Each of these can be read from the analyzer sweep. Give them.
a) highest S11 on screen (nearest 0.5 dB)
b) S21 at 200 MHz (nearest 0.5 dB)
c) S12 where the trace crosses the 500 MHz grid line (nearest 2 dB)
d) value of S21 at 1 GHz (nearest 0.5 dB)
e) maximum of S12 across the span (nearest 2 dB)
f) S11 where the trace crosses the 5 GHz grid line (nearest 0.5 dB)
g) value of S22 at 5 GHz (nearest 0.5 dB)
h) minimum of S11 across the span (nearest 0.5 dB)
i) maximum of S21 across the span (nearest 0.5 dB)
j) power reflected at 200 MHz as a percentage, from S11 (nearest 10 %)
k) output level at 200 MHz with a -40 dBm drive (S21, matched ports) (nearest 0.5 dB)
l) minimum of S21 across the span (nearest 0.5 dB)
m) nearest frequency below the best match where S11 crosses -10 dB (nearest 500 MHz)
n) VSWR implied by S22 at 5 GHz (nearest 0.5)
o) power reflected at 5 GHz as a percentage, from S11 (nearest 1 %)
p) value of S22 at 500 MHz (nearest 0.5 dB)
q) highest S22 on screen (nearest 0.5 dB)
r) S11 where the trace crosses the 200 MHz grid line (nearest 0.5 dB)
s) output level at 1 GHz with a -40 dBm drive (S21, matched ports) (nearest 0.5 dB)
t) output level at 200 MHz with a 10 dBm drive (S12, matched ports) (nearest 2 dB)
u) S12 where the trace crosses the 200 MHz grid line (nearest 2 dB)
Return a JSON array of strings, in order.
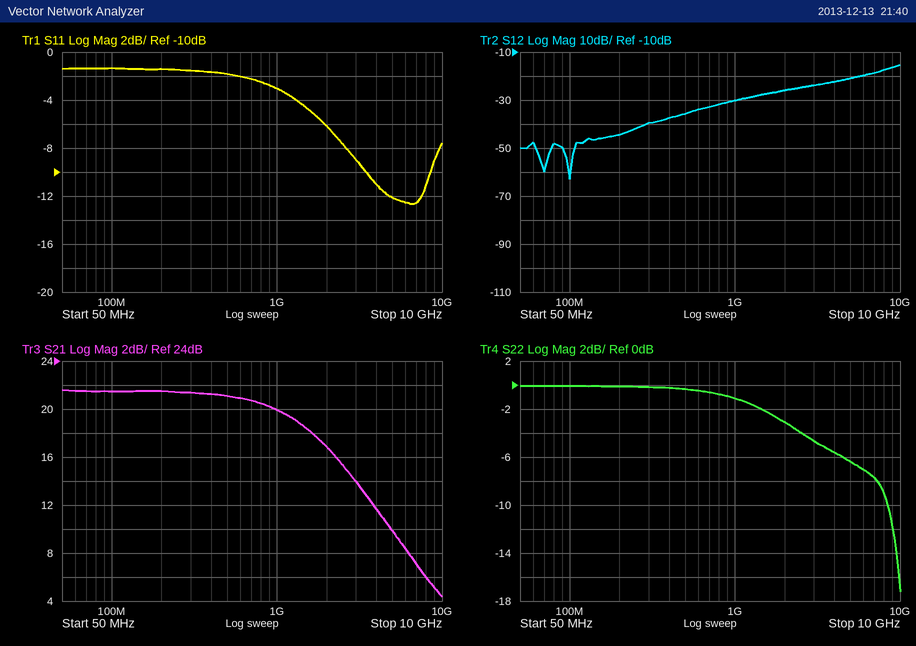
["-1.5 dB", "21.5 dB", "-36 dB", "20.0 dB", "-16 dB", "-12.0 dB", "-6.5 dB", "-12.5 dB", "21.5 dB", "70 %", "-18.5 dBm", "4.5 dB", "3.5 GHz", "3.0", "6 %", "-0.5 dB", "0.0 dB", "-1.5 dB", "-20.0 dBm", "-34 dBm", "-44 dB"]
